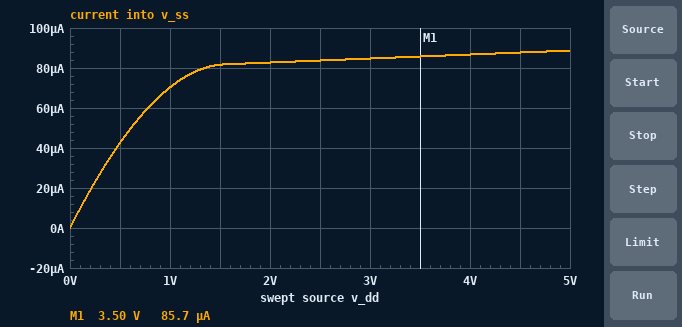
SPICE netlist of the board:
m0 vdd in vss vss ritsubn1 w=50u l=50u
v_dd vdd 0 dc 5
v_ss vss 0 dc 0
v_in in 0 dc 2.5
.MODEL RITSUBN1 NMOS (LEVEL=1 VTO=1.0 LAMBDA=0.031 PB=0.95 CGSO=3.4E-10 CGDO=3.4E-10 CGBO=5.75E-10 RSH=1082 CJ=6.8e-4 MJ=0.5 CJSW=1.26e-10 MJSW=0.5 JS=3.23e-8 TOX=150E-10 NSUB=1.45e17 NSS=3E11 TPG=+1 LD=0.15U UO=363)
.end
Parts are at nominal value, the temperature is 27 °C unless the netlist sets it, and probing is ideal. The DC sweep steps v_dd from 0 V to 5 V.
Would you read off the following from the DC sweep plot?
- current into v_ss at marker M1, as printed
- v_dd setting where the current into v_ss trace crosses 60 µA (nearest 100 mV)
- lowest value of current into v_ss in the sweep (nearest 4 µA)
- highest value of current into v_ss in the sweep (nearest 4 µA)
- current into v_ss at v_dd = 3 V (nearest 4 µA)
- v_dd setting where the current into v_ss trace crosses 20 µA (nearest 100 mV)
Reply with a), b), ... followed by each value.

a) 85.7 µA
b) 800 mV
c) 0 A
d) 88 µA
e) 84 µA
f) 200 mV
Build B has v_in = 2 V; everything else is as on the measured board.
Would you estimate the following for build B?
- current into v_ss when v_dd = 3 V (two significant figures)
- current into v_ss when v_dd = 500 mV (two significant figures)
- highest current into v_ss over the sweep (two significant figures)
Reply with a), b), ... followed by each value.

a) 40 µA
b) 28 µA
c) 42 µA
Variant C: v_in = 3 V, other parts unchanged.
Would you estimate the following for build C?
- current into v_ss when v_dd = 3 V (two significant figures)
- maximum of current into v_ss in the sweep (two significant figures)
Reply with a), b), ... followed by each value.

a) 140 µA
b) 150 µA
